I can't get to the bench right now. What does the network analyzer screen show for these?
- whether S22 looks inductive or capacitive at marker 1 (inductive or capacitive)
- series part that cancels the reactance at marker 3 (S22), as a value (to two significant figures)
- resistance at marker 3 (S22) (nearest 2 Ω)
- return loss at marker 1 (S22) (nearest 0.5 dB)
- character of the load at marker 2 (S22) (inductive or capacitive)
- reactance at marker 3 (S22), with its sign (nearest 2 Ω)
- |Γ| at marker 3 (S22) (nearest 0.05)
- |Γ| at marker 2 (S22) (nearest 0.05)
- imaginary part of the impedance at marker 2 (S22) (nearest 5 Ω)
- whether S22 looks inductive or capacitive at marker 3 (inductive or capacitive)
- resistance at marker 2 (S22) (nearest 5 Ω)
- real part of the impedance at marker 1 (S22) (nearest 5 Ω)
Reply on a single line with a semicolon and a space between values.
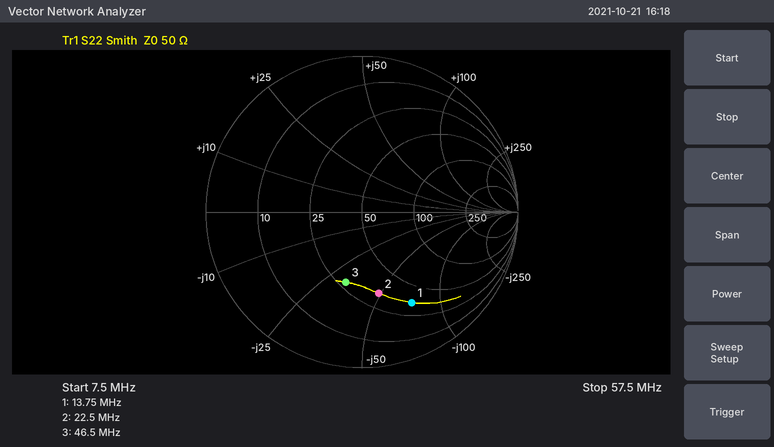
capacitive; 110 nH; 28 Ω; 3.5 dB; capacitive; -32 Ω; 0.45; 0.55; -50 Ω; capacitive; 35 Ω; 35 Ω
